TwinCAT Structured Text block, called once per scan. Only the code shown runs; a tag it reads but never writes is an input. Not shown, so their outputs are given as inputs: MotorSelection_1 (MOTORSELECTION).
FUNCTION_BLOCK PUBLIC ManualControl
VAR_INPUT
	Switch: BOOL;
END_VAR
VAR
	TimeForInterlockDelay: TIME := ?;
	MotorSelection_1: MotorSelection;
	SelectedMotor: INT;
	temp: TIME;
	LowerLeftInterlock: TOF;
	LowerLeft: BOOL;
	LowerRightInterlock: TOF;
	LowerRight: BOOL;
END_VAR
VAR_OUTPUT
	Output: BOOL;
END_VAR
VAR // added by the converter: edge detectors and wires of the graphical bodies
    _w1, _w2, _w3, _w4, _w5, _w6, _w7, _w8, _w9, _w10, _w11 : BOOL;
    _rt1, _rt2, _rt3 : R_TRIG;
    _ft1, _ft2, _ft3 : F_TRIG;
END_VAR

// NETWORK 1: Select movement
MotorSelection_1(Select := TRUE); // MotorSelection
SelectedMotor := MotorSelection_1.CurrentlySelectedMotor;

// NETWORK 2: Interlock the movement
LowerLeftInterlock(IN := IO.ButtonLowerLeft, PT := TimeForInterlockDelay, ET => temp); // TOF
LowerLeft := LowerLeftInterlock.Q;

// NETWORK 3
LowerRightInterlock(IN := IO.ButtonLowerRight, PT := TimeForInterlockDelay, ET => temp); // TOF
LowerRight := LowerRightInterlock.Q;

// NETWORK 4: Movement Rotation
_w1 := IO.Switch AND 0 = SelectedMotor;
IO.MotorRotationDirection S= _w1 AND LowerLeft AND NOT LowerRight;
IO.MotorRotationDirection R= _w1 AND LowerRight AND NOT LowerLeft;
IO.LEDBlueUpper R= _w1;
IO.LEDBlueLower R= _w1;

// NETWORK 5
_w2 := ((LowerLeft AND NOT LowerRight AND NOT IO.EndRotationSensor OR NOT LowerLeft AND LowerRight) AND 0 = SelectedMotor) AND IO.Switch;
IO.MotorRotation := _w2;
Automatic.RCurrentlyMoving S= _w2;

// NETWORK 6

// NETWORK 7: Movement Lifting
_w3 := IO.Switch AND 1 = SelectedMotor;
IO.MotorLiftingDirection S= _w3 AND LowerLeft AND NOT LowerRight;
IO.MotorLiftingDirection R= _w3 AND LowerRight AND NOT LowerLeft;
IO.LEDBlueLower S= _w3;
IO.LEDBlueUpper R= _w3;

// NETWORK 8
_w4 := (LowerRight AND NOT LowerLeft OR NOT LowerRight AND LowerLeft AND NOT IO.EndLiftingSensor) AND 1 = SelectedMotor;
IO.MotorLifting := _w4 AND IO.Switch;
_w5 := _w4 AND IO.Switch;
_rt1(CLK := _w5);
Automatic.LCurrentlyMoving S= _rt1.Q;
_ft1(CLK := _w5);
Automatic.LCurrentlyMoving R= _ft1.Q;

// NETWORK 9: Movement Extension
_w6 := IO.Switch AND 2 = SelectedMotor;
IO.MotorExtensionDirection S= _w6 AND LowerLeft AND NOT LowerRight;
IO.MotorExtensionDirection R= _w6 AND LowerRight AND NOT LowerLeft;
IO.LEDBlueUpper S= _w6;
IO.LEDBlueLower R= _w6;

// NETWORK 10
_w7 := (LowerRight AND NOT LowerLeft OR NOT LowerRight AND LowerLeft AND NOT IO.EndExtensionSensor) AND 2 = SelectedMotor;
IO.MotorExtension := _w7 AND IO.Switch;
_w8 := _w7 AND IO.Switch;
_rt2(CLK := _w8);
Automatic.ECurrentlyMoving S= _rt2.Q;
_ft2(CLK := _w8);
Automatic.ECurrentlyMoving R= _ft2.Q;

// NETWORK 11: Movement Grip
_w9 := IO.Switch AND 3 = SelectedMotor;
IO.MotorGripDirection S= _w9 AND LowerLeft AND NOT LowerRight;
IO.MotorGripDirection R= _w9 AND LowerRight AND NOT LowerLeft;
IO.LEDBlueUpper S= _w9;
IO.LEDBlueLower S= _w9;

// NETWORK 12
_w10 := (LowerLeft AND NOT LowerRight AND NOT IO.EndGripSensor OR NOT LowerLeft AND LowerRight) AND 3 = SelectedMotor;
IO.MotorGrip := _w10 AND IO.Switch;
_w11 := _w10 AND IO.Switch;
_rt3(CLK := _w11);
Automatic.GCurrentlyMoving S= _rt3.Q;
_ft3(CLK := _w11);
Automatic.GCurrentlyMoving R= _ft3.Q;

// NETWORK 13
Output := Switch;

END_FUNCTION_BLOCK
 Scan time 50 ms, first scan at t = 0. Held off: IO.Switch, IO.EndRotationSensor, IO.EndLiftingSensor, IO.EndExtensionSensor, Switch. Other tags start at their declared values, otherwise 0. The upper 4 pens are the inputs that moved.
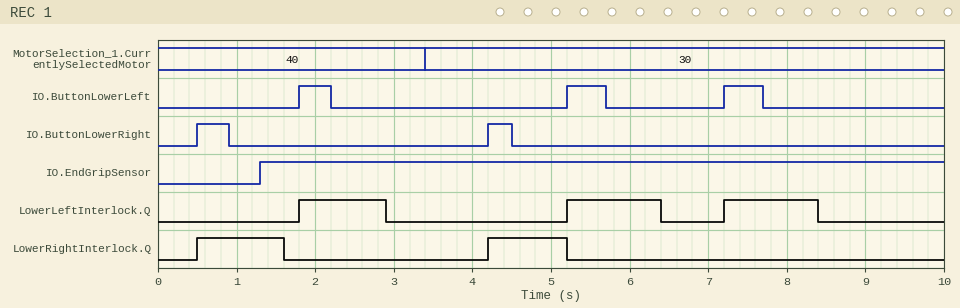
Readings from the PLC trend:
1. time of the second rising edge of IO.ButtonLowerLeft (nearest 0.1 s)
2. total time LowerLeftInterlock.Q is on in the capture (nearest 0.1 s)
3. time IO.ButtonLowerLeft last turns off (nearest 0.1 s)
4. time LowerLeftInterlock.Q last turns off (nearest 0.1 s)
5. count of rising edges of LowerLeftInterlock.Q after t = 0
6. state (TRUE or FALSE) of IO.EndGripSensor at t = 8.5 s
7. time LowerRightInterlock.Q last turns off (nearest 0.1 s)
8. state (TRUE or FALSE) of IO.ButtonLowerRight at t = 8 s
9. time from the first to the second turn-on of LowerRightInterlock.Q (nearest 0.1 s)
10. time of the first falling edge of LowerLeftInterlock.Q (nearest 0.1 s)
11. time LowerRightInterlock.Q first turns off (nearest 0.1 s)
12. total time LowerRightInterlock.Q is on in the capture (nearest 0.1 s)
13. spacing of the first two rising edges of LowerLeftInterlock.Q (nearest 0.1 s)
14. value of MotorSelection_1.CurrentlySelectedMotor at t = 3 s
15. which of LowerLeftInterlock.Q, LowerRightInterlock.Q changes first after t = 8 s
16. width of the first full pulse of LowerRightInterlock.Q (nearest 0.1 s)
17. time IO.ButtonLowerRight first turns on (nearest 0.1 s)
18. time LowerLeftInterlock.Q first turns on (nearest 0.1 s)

5.2 s
3.5 s
7.7 s
8.4 s
3
TRUE
5.2 s
FALSE
3.7 s
2.9 s
1.6 s
2.1 s
3.4 s
40
LowerLeftInterlock.Q
1.1 s
0.5 s
1.8 s
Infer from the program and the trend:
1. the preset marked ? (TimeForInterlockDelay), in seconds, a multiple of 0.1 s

0.7 s
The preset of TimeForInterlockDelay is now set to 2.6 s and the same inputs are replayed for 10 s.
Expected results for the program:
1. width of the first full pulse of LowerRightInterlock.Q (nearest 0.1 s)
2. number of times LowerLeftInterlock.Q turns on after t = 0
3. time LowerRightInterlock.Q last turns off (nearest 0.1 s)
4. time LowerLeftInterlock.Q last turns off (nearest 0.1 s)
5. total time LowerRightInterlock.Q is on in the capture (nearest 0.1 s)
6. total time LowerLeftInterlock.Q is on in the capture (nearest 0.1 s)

3.0 s
2
7.1 s
4.8 s
5.9 s
7.8 s
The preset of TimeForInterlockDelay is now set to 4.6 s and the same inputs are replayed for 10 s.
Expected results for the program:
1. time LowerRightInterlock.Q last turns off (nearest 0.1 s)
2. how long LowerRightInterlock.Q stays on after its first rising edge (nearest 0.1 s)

9.1 s
8.6 s
